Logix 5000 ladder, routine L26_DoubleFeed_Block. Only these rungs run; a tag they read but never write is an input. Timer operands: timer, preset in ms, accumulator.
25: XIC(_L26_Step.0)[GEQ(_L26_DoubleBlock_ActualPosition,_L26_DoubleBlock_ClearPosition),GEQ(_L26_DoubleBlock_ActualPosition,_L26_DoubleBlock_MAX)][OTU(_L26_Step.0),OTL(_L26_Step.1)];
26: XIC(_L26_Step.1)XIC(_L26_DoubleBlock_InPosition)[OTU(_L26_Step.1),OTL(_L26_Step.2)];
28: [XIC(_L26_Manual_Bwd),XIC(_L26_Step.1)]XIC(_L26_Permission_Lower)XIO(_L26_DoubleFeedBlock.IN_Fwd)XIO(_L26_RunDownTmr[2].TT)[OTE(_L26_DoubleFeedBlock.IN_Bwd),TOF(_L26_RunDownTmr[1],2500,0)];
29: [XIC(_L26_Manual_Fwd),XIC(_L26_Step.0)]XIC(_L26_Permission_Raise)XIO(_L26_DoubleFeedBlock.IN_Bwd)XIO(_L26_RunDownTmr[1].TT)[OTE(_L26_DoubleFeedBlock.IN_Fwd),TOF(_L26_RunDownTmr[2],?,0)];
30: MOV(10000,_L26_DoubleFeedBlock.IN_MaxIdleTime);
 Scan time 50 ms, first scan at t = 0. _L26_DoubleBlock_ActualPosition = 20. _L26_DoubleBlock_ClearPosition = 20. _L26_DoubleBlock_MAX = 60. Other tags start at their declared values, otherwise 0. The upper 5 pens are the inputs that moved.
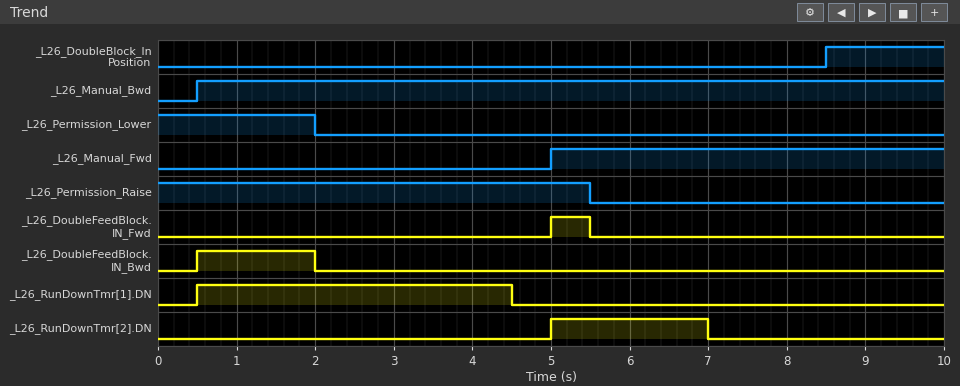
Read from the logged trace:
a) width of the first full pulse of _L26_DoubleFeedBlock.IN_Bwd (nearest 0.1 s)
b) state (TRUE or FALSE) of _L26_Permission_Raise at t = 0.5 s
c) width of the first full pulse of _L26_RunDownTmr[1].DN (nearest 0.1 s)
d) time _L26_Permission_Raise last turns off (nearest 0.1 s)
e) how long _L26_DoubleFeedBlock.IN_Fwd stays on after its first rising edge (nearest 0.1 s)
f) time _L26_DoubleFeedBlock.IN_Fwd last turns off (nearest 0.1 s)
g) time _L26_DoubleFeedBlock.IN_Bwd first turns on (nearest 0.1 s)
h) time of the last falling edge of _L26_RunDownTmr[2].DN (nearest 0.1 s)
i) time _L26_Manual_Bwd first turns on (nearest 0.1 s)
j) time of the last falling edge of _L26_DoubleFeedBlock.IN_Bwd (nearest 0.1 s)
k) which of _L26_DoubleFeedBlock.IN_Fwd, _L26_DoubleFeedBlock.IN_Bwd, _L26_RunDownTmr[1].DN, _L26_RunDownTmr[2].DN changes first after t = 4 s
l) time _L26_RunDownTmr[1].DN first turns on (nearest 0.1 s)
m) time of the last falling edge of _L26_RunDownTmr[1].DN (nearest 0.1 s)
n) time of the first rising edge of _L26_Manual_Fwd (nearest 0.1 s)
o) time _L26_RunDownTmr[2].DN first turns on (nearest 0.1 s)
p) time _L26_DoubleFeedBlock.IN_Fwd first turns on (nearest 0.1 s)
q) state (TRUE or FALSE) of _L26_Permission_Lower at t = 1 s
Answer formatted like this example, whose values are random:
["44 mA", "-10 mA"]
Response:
["1.5 s", "TRUE", "4.0 s", "5.5 s", "0.5 s", "5.5 s", "0.5 s", "7.0 s", "0.5 s", "2.0 s", "_L26_RunDownTmr[1].DN", "0.5 s", "4.5 s", "5.0 s", "5.0 s", "5.0 s", "TRUE"]
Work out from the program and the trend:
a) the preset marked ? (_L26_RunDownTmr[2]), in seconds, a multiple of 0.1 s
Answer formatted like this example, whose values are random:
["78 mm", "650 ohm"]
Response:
["1.5 s"]
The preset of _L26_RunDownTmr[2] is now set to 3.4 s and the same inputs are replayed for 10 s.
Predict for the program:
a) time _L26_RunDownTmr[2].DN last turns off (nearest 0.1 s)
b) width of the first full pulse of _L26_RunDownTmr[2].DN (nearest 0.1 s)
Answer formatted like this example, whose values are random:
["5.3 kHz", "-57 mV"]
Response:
["8.9 s", "3.9 s"]
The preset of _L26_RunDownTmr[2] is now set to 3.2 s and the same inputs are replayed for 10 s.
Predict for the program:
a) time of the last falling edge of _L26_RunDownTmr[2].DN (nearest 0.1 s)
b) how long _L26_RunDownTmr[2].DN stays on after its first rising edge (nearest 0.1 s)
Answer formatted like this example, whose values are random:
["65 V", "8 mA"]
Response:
["8.7 s", "3.7 s"]
